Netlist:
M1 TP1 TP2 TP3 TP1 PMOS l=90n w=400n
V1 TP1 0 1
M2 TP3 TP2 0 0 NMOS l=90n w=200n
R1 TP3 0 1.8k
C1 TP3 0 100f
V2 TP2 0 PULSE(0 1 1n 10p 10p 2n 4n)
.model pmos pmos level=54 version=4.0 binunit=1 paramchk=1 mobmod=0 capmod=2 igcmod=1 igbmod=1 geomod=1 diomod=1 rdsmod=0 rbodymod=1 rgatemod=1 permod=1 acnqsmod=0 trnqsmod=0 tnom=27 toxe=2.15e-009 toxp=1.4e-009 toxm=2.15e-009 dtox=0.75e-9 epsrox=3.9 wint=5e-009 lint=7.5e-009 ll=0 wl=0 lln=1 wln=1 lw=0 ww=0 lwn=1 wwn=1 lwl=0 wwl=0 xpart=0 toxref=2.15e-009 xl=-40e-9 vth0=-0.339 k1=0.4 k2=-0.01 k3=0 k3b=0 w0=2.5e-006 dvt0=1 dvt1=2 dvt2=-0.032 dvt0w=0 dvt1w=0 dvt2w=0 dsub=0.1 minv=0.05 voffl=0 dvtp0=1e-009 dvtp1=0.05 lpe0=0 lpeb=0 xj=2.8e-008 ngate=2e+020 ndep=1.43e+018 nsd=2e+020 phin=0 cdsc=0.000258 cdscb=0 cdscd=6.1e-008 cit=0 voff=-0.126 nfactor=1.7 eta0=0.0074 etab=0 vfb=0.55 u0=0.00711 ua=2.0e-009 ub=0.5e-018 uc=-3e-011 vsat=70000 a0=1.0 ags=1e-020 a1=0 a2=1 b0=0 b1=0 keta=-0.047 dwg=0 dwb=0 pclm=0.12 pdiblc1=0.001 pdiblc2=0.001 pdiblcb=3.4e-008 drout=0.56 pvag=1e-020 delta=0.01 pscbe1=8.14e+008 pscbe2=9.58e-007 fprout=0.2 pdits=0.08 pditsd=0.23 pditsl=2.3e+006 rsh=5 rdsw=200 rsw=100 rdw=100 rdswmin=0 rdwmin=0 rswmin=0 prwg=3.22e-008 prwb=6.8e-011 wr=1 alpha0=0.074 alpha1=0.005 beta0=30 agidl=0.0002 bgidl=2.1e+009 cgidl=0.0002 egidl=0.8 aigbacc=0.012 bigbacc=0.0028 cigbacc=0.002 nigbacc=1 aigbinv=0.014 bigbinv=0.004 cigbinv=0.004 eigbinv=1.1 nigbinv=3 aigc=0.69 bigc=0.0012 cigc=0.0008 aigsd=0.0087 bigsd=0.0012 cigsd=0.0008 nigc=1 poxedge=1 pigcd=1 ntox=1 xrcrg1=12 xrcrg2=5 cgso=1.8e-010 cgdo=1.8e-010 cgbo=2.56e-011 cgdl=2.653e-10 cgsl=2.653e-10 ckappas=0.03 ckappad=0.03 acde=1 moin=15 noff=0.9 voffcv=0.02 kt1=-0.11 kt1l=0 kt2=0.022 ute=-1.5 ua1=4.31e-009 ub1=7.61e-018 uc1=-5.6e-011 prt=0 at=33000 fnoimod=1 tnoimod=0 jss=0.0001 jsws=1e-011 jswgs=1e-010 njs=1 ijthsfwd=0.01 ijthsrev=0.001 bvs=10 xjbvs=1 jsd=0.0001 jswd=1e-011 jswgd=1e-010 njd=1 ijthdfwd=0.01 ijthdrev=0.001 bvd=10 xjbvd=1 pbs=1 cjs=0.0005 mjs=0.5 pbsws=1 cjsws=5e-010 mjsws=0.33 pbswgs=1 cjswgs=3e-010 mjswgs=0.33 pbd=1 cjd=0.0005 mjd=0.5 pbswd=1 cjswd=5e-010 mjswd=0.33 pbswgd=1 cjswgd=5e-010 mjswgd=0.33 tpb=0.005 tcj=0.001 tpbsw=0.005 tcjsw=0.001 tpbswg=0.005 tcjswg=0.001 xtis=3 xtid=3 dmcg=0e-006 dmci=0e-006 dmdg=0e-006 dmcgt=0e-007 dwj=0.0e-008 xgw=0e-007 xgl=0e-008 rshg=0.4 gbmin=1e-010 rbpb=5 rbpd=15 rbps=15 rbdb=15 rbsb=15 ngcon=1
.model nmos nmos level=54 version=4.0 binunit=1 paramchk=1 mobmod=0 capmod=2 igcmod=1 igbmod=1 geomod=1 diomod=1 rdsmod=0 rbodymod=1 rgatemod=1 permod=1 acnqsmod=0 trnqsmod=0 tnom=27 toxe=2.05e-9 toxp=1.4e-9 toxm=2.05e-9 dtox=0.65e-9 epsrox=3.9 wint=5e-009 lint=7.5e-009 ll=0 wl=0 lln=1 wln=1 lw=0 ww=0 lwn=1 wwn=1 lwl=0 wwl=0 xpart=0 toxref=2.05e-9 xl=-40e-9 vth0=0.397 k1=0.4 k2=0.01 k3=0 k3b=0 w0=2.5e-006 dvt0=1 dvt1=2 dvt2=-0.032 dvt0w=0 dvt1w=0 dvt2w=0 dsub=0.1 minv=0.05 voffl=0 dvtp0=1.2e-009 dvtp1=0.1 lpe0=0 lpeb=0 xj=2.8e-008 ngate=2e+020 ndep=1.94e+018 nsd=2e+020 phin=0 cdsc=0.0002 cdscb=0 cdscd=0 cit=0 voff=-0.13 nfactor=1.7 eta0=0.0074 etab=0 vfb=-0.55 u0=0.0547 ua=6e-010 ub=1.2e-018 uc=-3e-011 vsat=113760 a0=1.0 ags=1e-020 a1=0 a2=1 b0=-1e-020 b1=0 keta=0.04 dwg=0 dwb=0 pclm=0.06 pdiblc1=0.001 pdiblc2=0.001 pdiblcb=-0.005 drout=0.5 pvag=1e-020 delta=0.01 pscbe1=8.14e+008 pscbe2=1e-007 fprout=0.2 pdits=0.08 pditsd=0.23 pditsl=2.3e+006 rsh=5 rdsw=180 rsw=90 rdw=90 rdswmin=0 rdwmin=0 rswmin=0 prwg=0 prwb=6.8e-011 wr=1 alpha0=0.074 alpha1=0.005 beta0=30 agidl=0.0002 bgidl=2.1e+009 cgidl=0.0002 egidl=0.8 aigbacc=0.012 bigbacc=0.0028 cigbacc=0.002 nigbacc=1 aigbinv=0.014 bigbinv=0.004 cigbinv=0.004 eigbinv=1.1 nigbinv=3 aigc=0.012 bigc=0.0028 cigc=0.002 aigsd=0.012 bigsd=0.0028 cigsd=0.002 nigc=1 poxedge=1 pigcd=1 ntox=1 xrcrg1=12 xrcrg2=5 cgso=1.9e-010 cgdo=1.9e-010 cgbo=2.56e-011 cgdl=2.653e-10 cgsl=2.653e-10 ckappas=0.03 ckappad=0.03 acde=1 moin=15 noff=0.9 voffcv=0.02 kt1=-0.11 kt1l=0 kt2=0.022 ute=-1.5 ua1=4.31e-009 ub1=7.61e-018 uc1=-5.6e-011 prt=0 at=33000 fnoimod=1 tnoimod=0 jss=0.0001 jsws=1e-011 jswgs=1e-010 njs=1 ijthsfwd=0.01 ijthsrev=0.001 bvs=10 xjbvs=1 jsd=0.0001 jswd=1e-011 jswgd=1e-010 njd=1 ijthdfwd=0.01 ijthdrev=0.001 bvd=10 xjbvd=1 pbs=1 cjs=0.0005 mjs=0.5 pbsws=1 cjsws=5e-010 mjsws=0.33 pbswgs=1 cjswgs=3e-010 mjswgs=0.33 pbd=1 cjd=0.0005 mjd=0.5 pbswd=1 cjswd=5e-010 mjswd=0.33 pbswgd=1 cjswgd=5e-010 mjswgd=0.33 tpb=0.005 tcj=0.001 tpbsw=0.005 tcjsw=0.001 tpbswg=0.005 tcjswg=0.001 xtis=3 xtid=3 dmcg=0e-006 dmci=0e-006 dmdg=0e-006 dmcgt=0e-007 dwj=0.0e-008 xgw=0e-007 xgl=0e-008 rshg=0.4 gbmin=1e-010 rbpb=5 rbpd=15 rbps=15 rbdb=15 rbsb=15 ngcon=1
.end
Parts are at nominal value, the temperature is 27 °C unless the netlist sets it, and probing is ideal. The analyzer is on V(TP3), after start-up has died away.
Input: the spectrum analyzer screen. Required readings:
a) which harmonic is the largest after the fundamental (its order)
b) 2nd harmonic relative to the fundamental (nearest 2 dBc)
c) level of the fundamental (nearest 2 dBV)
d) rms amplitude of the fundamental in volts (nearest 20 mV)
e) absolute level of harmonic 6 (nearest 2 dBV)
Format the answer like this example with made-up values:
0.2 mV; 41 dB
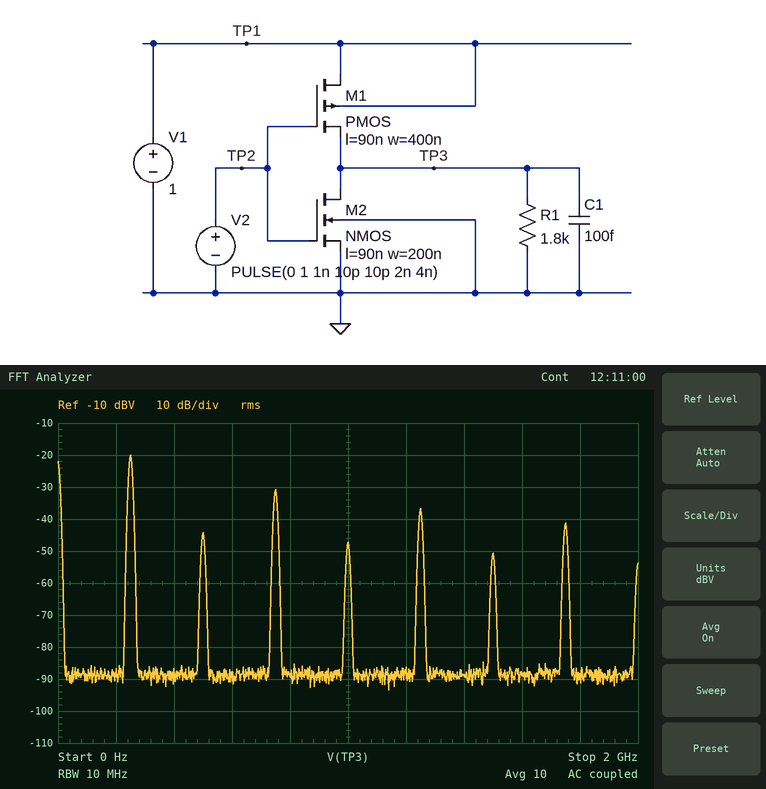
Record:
3; -24 dBc; -20 dBV; 100 mV; -50 dBV
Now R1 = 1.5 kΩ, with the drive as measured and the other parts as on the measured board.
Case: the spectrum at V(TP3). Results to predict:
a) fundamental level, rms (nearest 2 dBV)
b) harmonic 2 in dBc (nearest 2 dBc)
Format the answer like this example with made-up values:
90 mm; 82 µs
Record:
-22 dBV; -26 dBc
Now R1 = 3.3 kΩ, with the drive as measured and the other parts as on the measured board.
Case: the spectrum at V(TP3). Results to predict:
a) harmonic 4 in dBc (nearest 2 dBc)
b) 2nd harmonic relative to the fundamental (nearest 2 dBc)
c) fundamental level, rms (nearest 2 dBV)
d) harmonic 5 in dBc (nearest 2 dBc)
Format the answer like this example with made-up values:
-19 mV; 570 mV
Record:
-26 dBc; -20 dBc; -16 dBV; -18 dBc
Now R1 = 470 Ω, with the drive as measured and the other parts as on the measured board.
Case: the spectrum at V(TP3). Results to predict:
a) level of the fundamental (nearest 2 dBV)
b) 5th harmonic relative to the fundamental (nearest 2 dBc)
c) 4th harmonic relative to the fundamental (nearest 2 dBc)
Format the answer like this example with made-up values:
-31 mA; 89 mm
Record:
-30 dBV; -14 dBc; -36 dBc
